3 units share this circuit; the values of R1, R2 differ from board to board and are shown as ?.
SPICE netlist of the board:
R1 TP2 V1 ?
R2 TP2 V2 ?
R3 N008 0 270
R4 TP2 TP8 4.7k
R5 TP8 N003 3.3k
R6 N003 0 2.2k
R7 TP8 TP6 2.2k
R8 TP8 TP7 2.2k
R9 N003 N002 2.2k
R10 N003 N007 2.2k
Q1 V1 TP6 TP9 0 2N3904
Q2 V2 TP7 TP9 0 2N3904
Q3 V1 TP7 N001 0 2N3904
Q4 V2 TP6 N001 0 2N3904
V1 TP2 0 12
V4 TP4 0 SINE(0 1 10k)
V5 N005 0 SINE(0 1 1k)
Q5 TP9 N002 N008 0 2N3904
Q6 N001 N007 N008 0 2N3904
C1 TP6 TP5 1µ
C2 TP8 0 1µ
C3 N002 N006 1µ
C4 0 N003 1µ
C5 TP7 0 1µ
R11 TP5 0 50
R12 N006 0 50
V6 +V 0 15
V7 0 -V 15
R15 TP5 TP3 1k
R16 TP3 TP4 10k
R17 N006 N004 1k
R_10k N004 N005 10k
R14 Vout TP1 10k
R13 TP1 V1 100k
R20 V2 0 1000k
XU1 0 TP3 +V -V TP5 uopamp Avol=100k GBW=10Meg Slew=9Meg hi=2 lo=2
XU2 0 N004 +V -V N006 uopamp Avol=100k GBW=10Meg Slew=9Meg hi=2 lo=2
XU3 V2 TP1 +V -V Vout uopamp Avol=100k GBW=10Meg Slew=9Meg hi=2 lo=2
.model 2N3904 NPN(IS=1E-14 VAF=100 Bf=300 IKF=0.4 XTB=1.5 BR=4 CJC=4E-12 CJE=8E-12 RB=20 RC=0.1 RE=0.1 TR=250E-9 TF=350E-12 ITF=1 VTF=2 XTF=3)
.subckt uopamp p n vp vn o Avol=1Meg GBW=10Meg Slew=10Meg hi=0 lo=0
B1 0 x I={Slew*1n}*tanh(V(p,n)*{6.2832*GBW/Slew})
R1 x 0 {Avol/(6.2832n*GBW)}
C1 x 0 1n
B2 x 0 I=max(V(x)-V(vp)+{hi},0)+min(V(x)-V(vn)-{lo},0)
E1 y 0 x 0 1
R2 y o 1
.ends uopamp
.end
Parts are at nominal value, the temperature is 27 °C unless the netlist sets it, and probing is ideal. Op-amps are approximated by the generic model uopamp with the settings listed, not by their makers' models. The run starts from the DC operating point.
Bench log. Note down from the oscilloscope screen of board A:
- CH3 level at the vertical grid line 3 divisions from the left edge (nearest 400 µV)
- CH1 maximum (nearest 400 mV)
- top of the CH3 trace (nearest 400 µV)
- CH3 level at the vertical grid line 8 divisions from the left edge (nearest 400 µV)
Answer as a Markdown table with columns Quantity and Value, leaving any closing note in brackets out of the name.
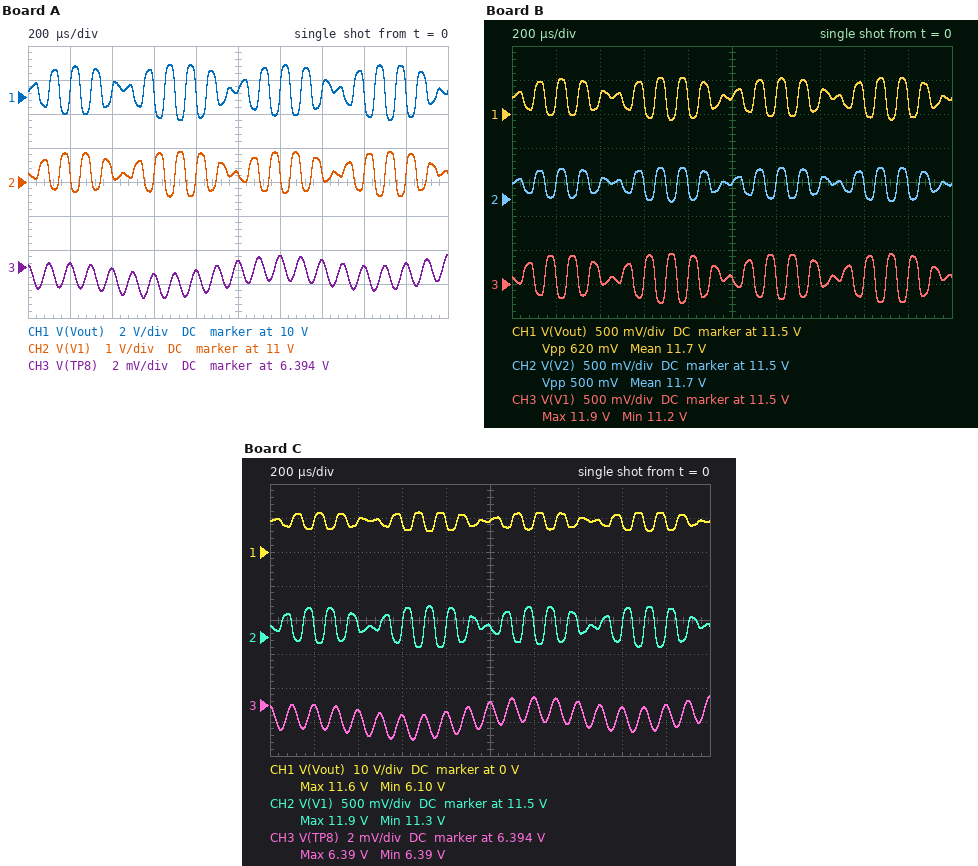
| Quantity | Value |
|---|---|
| CH3 level at the vertical grid line 3 divisions from the left edge | 6.3936 V |
| CH1 maximum | 12.0 V |
| top of the CH3 trace | 6.3948 V |
| CH3 level at the vertical grid line 8 divisions from the left edge | 6.3940 V |
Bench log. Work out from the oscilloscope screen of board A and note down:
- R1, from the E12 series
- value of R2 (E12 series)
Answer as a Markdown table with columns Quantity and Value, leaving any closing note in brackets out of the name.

| Quantity | Value |
|---|---|
| R1, from the E12 series | 220 Ω |
| value of R2 | 470 Ω |
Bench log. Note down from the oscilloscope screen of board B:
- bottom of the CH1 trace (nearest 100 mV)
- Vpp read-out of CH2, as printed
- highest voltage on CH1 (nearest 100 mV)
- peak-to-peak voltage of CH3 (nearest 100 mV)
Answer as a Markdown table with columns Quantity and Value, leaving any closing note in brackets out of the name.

| Quantity | Value |
|---|---|
| bottom of the CH1 trace | 11.4 V |
| Vpp read-out of CH2, as printed | 500 mV |
| highest voltage on CH1 | 12.0 V |
| peak-to-peak voltage of CH3 | 700 mV |
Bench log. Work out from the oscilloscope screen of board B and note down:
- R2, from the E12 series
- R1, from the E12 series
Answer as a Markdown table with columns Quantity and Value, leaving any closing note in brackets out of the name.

| Quantity | Value |
|---|---|
| R2, from the E12 series | 82 Ω |
| R1, from the E12 series | 120 Ω |
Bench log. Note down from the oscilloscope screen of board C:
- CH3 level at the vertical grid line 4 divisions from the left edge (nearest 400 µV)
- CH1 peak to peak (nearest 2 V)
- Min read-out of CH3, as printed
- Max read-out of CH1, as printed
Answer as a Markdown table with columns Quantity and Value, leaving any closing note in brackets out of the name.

| Quantity | Value |
|---|---|
| CH3 level at the vertical grid line 4 divisions from the left edge | 6.3936 V |
| CH1 peak to peak | 6 V |
| Min read-out of CH3, as printed | 6.39 V |
| Max read-out of CH1, as printed | 11.6 V |
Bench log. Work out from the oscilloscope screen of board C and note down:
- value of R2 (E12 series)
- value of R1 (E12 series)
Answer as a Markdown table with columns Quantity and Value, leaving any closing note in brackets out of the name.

| Quantity | Value |
|---|---|
| value of R2 | 820 Ω |
| value of R1 | 100 Ω |
